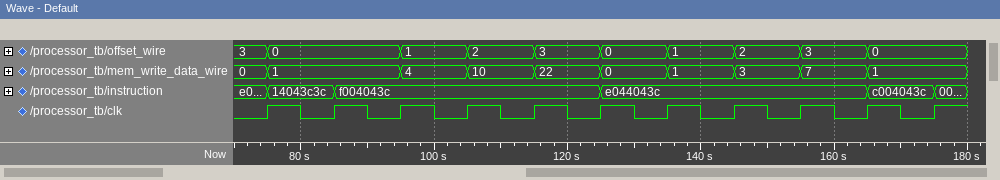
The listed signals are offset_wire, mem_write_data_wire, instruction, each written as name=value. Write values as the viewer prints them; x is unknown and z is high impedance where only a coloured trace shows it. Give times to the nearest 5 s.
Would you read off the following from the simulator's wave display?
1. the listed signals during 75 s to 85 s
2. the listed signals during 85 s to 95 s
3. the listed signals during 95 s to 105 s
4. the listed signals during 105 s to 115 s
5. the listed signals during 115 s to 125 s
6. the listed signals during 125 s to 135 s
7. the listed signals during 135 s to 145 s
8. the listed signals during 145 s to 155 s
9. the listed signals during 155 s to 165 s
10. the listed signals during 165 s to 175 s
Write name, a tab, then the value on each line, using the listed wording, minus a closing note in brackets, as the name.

the listed signals during 75 s to 85 s	offset_wire=0, mem_write_data_wire=1, instruction=14043c3c
the listed signals during 85 s to 95 s	offset_wire=0, mem_write_data_wire=1, instruction=f004043c
the listed signals during 95 s to 105 s	offset_wire=1, mem_write_data_wire=4, instruction=f004043c
the listed signals during 105 s to 115 s	offset_wire=2, mem_write_data_wire=10, instruction=f004043c
the listed signals during 115 s to 125 s	offset_wire=3, mem_write_data_wire=22, instruction=f004043c
the listed signals during 125 s to 135 s	offset_wire=0, mem_write_data_wire=0, instruction=e044043c
the listed signals during 135 s to 145 s	offset_wire=1, mem_write_data_wire=1, instruction=e044043c
the listed signals during 145 s to 155 s	offset_wire=2, mem_write_data_wire=3, instruction=e044043c
the listed signals during 155 s to 165 s	offset_wire=3, mem_write_data_wire=7, instruction=e044043c
the listed signals during 165 s to 175 s	offset_wire=0, mem_write_data_wire=1, instruction=c004043c
